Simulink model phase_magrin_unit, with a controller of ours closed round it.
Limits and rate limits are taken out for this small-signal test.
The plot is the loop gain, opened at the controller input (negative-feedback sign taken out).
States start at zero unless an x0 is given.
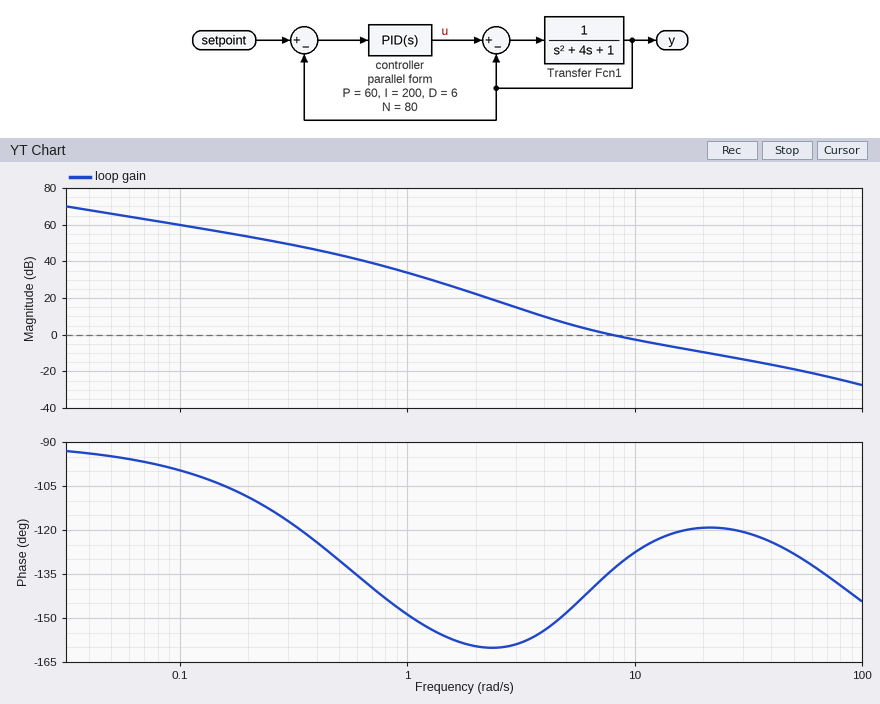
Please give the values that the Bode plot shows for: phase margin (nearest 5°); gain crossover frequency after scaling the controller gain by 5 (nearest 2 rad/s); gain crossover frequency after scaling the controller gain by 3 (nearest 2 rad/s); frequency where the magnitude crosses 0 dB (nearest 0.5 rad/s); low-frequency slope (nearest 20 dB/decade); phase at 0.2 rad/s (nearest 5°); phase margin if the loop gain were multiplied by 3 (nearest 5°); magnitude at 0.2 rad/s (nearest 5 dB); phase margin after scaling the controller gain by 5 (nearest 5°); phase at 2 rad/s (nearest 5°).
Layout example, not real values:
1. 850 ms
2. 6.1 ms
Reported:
1. 45°
2. 32 rad/s
3. 20 rad/s
4. 8.0 rad/s
5. -20 dB/decade
6. -110°
7. 60°
8. 55 dB
9. 60°
10. -160°
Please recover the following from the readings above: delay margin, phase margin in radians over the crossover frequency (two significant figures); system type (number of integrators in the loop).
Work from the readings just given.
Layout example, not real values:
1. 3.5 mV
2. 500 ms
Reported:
1. 0.098 s
2. 1
